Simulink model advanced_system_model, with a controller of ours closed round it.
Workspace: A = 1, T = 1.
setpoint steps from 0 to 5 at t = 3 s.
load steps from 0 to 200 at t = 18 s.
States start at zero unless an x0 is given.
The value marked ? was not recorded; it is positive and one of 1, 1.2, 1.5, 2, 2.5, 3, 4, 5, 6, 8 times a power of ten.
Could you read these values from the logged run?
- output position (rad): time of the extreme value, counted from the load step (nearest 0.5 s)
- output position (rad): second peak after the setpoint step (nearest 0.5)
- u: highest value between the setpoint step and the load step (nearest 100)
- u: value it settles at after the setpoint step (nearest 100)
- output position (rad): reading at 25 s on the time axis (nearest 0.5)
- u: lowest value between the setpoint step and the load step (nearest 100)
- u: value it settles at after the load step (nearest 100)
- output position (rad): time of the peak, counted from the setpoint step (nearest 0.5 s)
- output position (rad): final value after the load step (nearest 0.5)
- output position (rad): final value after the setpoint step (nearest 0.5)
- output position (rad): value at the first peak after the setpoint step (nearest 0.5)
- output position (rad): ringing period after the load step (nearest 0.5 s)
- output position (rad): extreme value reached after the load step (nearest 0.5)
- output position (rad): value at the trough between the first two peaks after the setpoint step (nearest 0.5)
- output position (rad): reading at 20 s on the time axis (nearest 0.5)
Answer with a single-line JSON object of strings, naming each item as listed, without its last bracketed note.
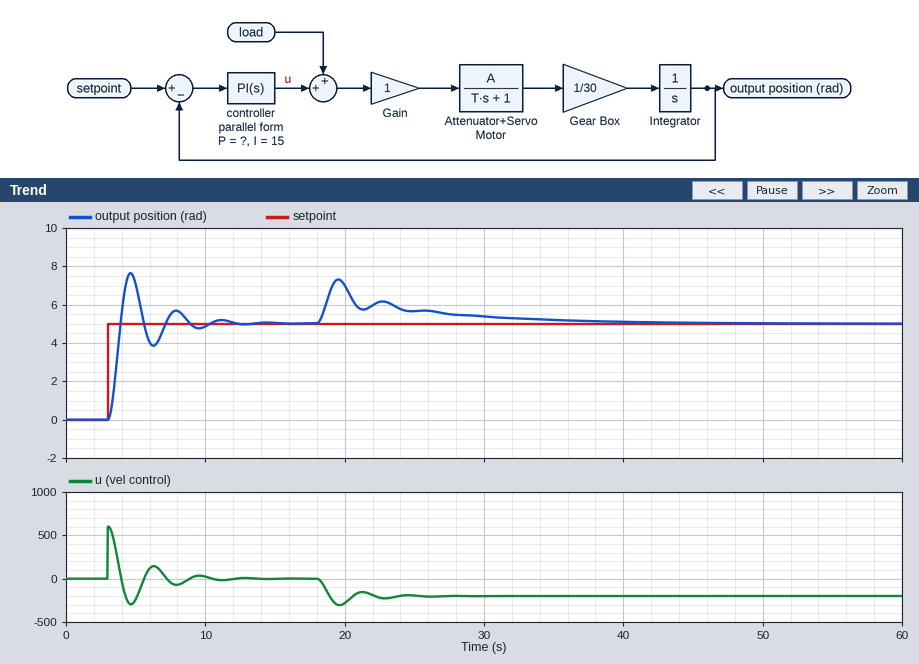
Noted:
{"output position (rad): time of the extreme value, counted from the load step": "1.5 s", "output position (rad): second peak after the setpoint step": "5.5", "u: highest value between the setpoint step and the load step": "600", "u: value it settles at after the setpoint step": "0", "output position (rad): reading at 25 s on the time axis": "5.5", "u: lowest value between the setpoint step and the load step": "-300", "u: value it settles at after the load step": "-200", "output position (rad): time of the peak, counted from the setpoint step": "1.5 s", "output position (rad): final value after the load step": "5.0", "output position (rad): final value after the setpoint step": "5.0", "output position (rad): value at the first peak after the setpoint step": "7.5", "output position (rad): ringing period after the load step": "3.0 s", "output position (rad): extreme value reached after the load step": "7.5", "output position (rad): value at the trough between the first two peaks after the setpoint step": "4.0", "output position (rad): reading at 20 s on the time axis": "7.0"}
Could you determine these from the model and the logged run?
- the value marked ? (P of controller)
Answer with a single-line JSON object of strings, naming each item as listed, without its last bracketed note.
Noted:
{"the value marked ?": "120"}
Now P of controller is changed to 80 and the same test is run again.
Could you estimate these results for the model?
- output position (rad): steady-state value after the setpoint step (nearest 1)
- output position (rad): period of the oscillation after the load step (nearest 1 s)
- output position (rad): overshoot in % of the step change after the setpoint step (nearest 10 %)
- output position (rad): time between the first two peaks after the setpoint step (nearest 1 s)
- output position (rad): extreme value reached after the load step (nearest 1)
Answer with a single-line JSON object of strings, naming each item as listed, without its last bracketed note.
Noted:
{"output position (rad): steady-state value after the setpoint step": "5", "output position (rad): period of the oscillation after the load step": "4 s", "output position (rad): overshoot in % of the step change after the setpoint step": "50 %", "output position (rad): time between the first two peaks after the setpoint step": "4 s", "output position (rad): extreme value reached after the load step": "8"}
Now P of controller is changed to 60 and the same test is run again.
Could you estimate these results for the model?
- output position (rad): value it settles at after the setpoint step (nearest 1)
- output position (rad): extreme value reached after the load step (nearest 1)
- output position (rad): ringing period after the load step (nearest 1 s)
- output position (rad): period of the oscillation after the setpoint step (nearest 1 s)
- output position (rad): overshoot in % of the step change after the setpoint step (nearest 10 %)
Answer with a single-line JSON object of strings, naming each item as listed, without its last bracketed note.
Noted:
{"output position (rad): value it settles at after the setpoint step": "5", "output position (rad): extreme value reached after the load step": "9", "output position (rad): ringing period after the load step": "5 s", "output position (rad): period of the oscillation after the setpoint step": "5 s", "output position (rad): overshoot in % of the step change after the setpoint step": "50 %"}
